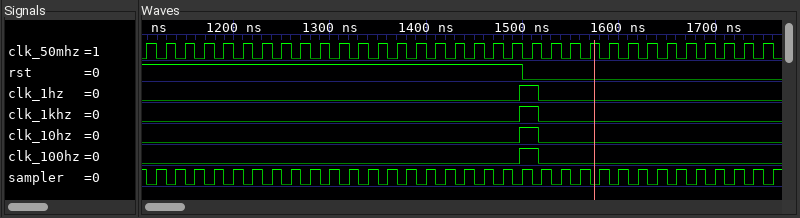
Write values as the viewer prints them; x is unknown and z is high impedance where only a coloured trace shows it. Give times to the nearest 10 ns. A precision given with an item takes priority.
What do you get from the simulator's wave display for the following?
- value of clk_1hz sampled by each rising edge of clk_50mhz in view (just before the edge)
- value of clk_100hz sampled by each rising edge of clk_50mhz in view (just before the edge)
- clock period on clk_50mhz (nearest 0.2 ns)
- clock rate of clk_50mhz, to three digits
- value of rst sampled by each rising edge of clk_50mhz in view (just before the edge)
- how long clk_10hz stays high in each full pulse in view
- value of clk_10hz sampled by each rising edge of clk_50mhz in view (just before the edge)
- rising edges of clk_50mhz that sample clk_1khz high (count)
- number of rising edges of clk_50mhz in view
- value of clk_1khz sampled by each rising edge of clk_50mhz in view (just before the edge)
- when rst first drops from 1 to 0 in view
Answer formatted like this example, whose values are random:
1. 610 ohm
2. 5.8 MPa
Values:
1. 0 0 0 0 0 0 0 0 0 0 0 0 0 0 0 0 0 0 0 0 1 0 0 0 0 0 0 0 0 0 0 0 0
2. 0 0 0 0 0 0 0 0 0 0 0 0 0 0 0 0 0 0 0 0 1 0 0 0 0 0 0 0 0 0 0 0 0
3. 20 ns
4. 50.0 MHz
5. 1 1 1 1 1 1 1 1 1 1 1 1 1 1 1 1 1 1 1 1 0 0 0 0 0 0 0 0 0 0 0 0 0
6. 20 ns
7. 0 0 0 0 0 0 0 0 0 0 0 0 0 0 0 0 0 0 0 0 1 0 0 0 0 0 0 0 0 0 0 0 0
8. 1
9. 33
10. 0 0 0 0 0 0 0 0 0 0 0 0 0 0 0 0 0 0 0 0 1 0 0 0 0 0 0 0 0 0 0 0 0
11. 1500 ns
